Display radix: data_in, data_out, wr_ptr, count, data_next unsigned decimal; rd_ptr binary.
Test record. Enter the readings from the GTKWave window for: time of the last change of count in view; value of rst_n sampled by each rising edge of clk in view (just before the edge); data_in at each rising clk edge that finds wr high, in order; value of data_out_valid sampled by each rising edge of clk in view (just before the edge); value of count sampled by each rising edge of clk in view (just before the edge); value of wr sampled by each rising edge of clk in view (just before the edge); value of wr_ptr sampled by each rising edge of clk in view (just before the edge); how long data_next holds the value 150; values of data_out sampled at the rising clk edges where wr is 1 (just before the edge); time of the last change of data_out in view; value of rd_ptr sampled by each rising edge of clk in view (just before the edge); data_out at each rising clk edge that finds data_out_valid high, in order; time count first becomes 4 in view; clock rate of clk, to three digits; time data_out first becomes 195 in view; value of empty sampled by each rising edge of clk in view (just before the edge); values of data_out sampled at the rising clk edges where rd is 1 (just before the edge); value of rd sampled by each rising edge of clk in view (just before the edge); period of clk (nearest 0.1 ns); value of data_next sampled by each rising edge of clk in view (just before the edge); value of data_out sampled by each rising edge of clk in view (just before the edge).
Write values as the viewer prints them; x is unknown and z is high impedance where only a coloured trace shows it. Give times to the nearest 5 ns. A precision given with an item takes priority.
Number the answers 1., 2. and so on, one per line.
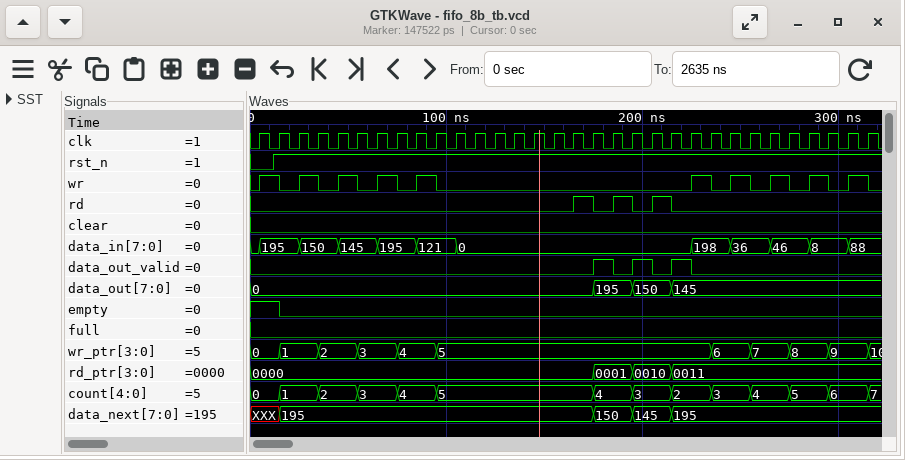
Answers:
1. 315 ns
2. 0 1 1 1 1 1 1 1 1 1 1 1 1 1 1 1 1 1 1 1 1 1 1 1 1 1 1 1 1 1 1 1
3. 195, 150, 145, 195, 121, 198, 36, 46, 8, 88
4. 0 0 0 0 0 0 0 0 0 0 0 0 0 0 0 0 0 0 1 0 1 0 1 0 0 0 0 0 0 0 0 0
5. 0, 0, 1, 1, 2, 2, 3, 3, 4, 4, 5, 5, 5, 5, 5, 5, 5, 5, 4, 4, 3, 3, 2, 2, 3, 3, 4, 4, 5, 5, 6, 6
6. 0 1 0 1 0 1 0 1 0 1 0 0 0 0 0 0 0 0 0 0 0 0 0 1 0 1 0 1 0 1 0 1
7. 0, 0, 1, 1, 2, 2, 3, 3, 4, 4, 5, 5, 5, 5, 5, 5, 5, 5, 5, 5, 5, 5, 5, 5, 6, 6, 7, 7, 8, 8, 9, 9
8. 20 ns
9. 0, 0, 0, 0, 0, 145, 145, 145, 145, 145
10. 215 ns
11. 0000, 0000, 0000, 0000, 0000, 0000, 0000, 0000, 0000, 0000, 0000, 0000, 0000, 0000, 0000, 0000, 0000, 0000, 0001, 0001, 0010, 0010, 0011, 0011, 0011, 0011, 0011, 0011, 0011, 0011, 0011, 0011
12. 195, 150, 145
13. 75 ns
14. 100 MHz
15. 175 ns
16. 1 1 0 0 0 0 0 0 0 0 0 0 0 0 0 0 0 0 0 0 0 0 0 0 0 0 0 0 0 0 0 0
17. 0, 195, 150
18. 0 0 0 0 0 0 0 0 0 0 0 0 0 0 0 0 0 1 0 1 0 1 0 0 0 0 0 0 0 0 0 0
19. 10 ns
20. XXX, XXX, 195, 195, 195, 195, 195, 195, 195, 195, 195, 195, 195, 195, 195, 195, 195, 195, 150, 150, 145, 145, 195, 195, 195, 195, 195, 195, 195, 195, 195, 195
21. 0, 0, 0, 0, 0, 0, 0, 0, 0, 0, 0, 0, 0, 0, 0, 0, 0, 0, 195, 195, 150, 150, 145, 145, 145, 145, 145, 145, 145, 145, 145, 145
